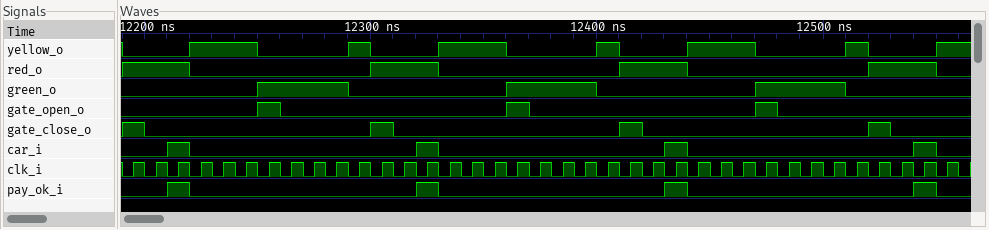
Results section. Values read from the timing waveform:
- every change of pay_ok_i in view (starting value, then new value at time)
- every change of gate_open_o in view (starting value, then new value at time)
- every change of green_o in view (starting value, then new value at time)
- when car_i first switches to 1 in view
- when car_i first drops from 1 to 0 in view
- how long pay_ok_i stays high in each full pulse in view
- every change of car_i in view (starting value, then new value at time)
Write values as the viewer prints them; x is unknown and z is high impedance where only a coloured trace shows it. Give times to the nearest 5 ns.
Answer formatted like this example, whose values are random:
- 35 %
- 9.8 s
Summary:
- 0, 1 at 12210 ns, 0 at 12220 ns, 1 at 12320 ns, 0 at 12330 ns, 1 at 12430 ns, 0 at 12440 ns, 1 at 12540 ns, 0 at 12550 ns
- 0, 1 at 12250 ns, 0 at 12260 ns, 1 at 12360 ns, 0 at 12370 ns, 1 at 12470 ns, 0 at 12480 ns
- 0, 1 at 12250 ns, 0 at 12290 ns, 1 at 12360 ns, 0 at 12400 ns, 1 at 12470 ns, 0 at 12510 ns
- 12210 ns
- 12220 ns
- 10 ns, 10 ns, 10 ns, 10 ns
- 0, 1 at 12210 ns, 0 at 12220 ns, 1 at 12320 ns, 0 at 12330 ns, 1 at 12430 ns, 0 at 12440 ns, 1 at 12540 ns, 0 at 12550 ns
